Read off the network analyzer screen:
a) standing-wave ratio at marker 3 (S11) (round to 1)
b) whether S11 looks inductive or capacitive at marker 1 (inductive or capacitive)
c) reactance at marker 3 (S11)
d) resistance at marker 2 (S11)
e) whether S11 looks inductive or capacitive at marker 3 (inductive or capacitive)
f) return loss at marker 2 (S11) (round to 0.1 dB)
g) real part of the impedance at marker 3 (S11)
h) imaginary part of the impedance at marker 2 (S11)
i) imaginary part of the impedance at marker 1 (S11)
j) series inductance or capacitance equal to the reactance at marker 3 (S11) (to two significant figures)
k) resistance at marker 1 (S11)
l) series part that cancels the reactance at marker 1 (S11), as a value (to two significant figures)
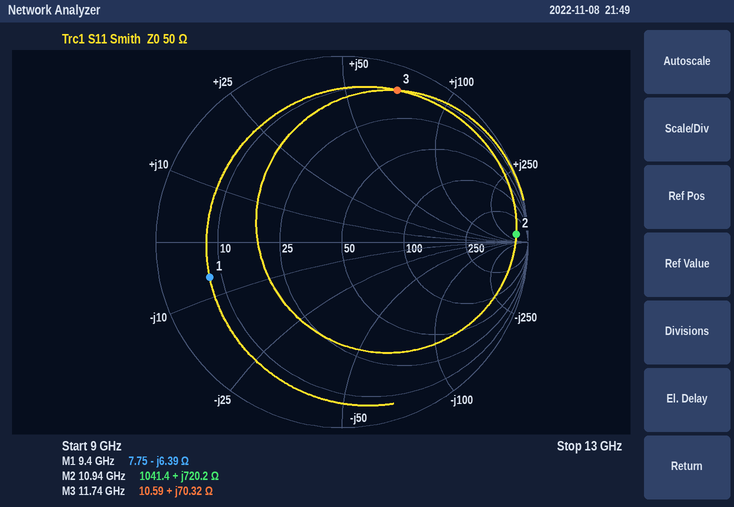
14
capacitive
+70.32 Ω
1041.4 Ω
inductive
0.6 dB
10.59 Ω
+720.2 Ω
-6.39 Ω
950 pH
7.75 Ω
110 pH
